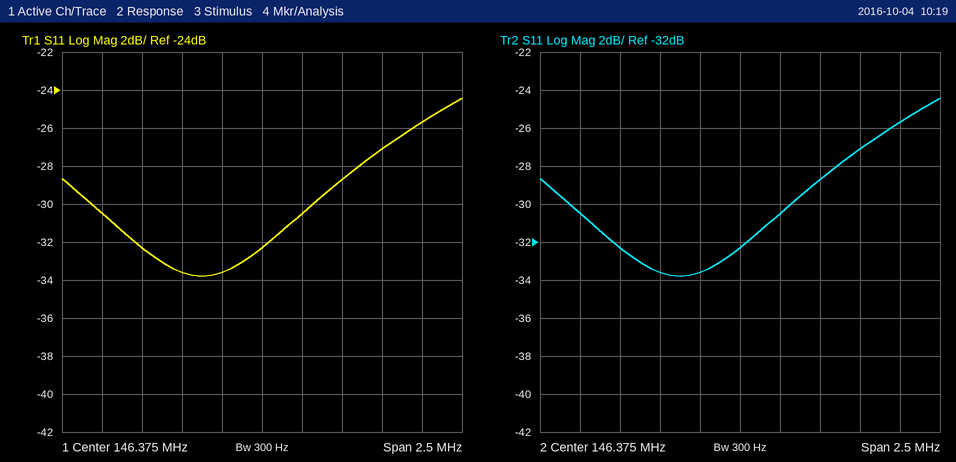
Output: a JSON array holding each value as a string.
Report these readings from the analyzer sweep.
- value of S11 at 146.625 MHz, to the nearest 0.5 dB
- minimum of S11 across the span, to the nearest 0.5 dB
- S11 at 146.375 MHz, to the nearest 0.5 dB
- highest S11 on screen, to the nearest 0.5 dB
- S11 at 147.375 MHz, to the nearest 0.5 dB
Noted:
["-30.5 dB", "-34.0 dB", "-32.5 dB", "-24.5 dB", "-25.5 dB"]
